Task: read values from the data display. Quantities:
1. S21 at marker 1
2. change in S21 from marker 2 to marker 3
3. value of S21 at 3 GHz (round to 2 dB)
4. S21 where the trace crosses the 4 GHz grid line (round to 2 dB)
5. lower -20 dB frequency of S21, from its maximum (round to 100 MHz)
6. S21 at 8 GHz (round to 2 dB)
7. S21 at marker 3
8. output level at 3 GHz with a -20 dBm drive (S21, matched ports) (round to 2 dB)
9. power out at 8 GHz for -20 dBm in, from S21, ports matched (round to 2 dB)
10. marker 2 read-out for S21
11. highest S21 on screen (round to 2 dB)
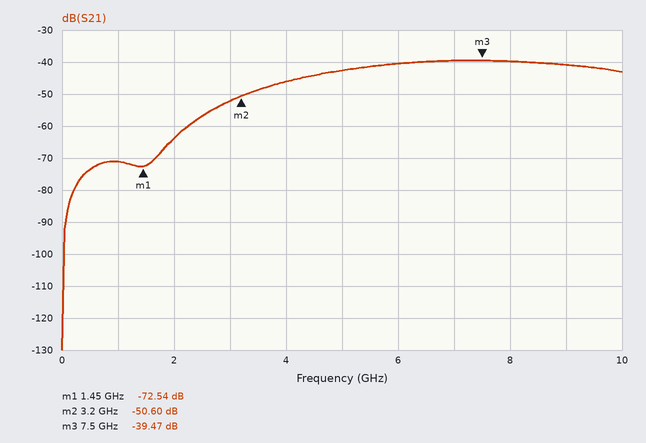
-72.54 dB
11.13 dB
-52 dB
-46 dB
2.3 GHz
-40 dB
-39.47 dB
-72 dBm
-60 dBm
-50.60 dB
-40 dB
